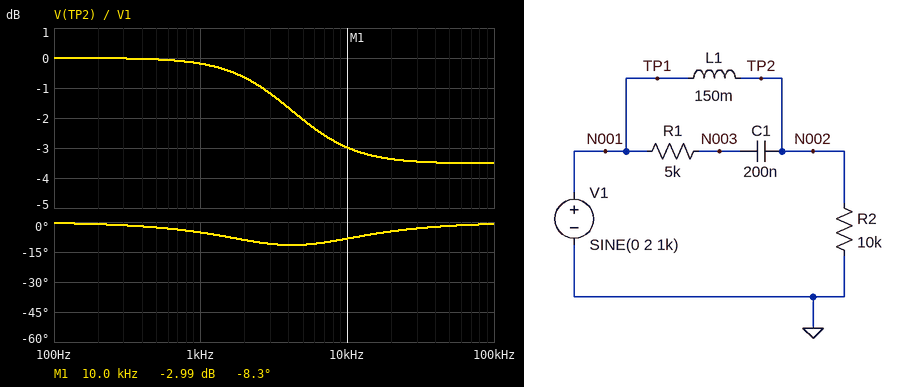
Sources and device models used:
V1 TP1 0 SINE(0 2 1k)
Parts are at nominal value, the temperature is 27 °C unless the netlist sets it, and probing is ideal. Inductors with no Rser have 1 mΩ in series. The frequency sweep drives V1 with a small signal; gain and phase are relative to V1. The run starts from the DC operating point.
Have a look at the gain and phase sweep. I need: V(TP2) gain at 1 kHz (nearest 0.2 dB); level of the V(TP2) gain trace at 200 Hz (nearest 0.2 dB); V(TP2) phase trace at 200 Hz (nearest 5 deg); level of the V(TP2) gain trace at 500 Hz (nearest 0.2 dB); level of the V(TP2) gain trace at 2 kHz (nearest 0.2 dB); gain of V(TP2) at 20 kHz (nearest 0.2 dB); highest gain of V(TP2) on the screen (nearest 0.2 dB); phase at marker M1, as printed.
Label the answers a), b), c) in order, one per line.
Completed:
a) -0.2 dB
b) 0 dB
c) 0 deg
d) 0 dB
e) -0.6 dB
f) -3.4 dB
g) 0 dB
h) -8.3 deg
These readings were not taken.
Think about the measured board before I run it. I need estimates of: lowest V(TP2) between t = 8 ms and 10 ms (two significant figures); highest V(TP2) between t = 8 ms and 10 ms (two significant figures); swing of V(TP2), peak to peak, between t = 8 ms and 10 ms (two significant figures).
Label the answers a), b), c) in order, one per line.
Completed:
a) -2.0 V
b) 2.0 V
c) 3.9 V
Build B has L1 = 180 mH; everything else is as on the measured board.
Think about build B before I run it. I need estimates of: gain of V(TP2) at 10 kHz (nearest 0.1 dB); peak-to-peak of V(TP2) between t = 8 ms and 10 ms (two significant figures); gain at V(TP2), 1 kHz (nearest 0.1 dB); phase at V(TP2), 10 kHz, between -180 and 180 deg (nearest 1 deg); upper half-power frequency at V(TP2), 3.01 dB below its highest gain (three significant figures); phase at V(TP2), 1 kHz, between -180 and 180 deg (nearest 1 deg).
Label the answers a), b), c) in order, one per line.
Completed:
a) -3.1 dB
b) 3.9 V
c) -0.3 dB
d) -7 deg
e) 8.52 kHz
f) -6 deg
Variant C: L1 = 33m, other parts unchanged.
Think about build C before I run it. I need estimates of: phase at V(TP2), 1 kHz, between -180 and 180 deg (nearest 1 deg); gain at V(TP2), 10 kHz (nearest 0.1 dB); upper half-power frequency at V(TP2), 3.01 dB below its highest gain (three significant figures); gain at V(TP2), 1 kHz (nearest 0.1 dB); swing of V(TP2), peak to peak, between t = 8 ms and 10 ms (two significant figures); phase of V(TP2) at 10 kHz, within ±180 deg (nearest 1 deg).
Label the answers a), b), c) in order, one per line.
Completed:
a) -1 deg
b) -0.7 dB
c) 47.9 kHz
d) 0 dB
e) 4.0 V
f) -9 deg
